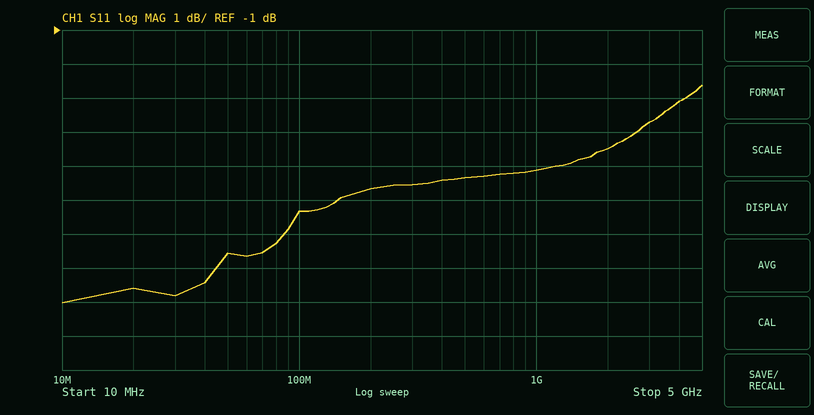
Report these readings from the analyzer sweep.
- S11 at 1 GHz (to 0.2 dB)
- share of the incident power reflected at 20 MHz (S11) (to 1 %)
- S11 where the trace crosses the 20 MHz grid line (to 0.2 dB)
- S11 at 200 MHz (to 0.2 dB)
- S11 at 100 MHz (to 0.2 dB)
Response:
-5.2 dB
14 %
-8.6 dB
-5.6 dB
-6.4 dB
